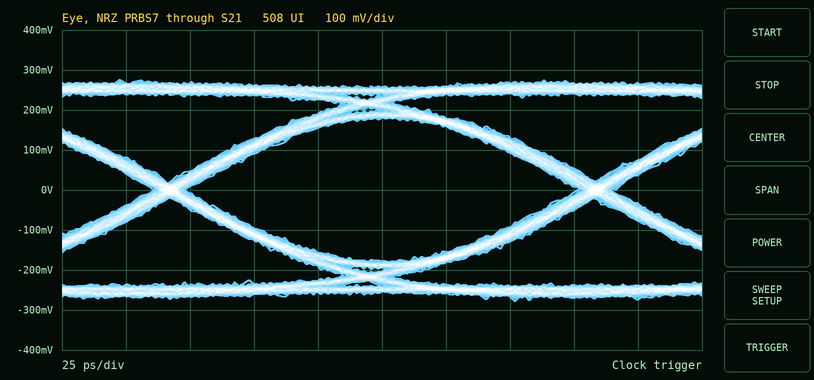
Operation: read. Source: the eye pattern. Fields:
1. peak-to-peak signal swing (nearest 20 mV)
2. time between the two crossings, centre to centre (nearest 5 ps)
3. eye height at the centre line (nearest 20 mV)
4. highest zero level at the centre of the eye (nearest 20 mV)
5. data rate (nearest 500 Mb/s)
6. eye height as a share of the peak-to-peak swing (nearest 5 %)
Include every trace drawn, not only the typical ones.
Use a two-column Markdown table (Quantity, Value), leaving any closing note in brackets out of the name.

| Quantity | Value |
|---|---|
| peak-to-peak signal swing | 560 mV |
| time between the two crossings, centre to centre | 165 ps |
| eye height at the centre line | 360 mV |
| highest zero level at the centre of the eye | -180 mV |
| data rate | 6.0 Gb/s |
| eye height as a share of the peak-to-peak swing | 65 % |
